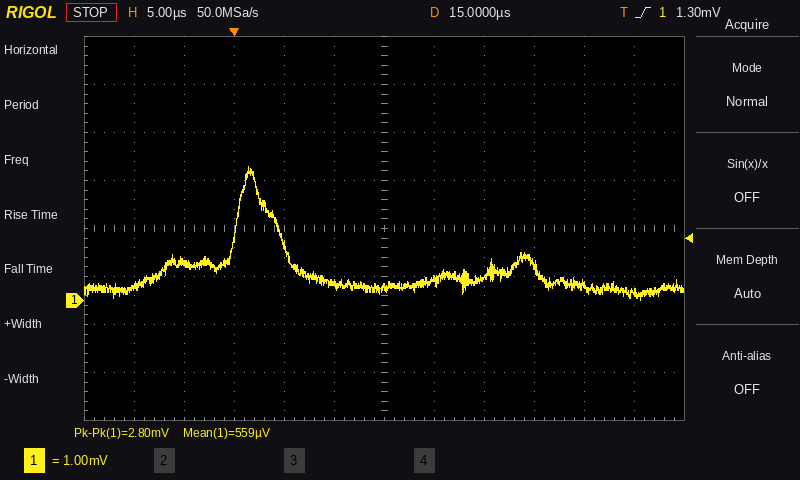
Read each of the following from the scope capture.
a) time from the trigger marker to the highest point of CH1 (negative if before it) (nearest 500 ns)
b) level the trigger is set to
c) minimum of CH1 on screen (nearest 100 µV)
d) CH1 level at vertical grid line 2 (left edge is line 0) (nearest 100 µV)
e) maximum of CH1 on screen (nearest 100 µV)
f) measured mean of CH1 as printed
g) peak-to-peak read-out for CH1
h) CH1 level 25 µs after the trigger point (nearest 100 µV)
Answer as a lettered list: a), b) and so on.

a) +1.5 µs
b) 1.30 mV
c) 0.0 mV
d) 800 µV
e) 2.8 mV
f) 559 µV
g) 2.80 mV
h) 500 µV
